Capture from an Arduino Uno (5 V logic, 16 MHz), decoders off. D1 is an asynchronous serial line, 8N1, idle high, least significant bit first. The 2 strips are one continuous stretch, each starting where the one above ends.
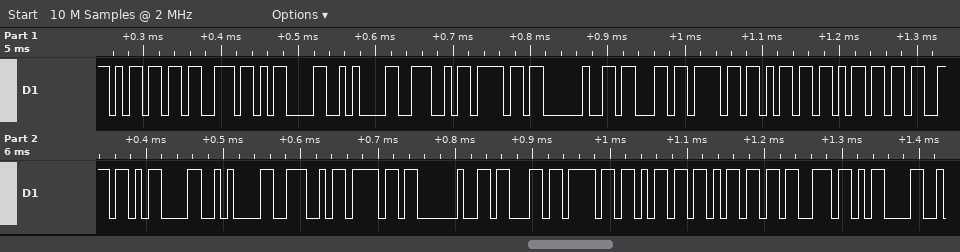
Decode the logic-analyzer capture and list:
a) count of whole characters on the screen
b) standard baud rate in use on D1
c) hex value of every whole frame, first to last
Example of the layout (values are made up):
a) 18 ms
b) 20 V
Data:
a) 23
b) 115200 baud
c) 0x6D 0x73 0x0D 0x0A 0x4E 0x6F 0x20 0x63 0x6F 0x6D 0x6D 0x73 0x0D 0x0A 0x4E 0x6F 0x20 0x63 0x6F 0x6D 0x6D 0x73 0x0D
